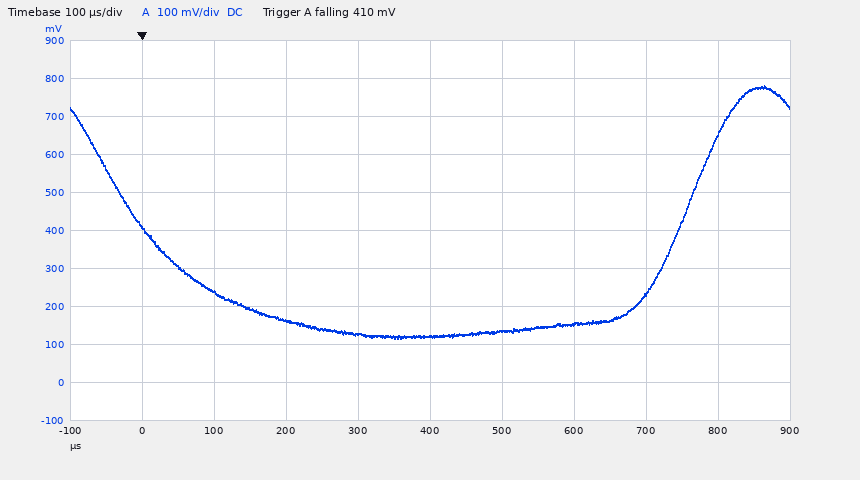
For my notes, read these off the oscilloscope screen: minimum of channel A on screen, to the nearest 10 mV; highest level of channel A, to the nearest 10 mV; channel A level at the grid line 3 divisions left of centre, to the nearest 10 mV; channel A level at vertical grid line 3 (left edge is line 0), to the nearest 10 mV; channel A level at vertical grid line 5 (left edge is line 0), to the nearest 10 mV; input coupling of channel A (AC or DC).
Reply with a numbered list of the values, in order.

1. 120 mV
2. 780 mV
3. 240 mV
4. 160 mV
5. 120 mV
6. DC
